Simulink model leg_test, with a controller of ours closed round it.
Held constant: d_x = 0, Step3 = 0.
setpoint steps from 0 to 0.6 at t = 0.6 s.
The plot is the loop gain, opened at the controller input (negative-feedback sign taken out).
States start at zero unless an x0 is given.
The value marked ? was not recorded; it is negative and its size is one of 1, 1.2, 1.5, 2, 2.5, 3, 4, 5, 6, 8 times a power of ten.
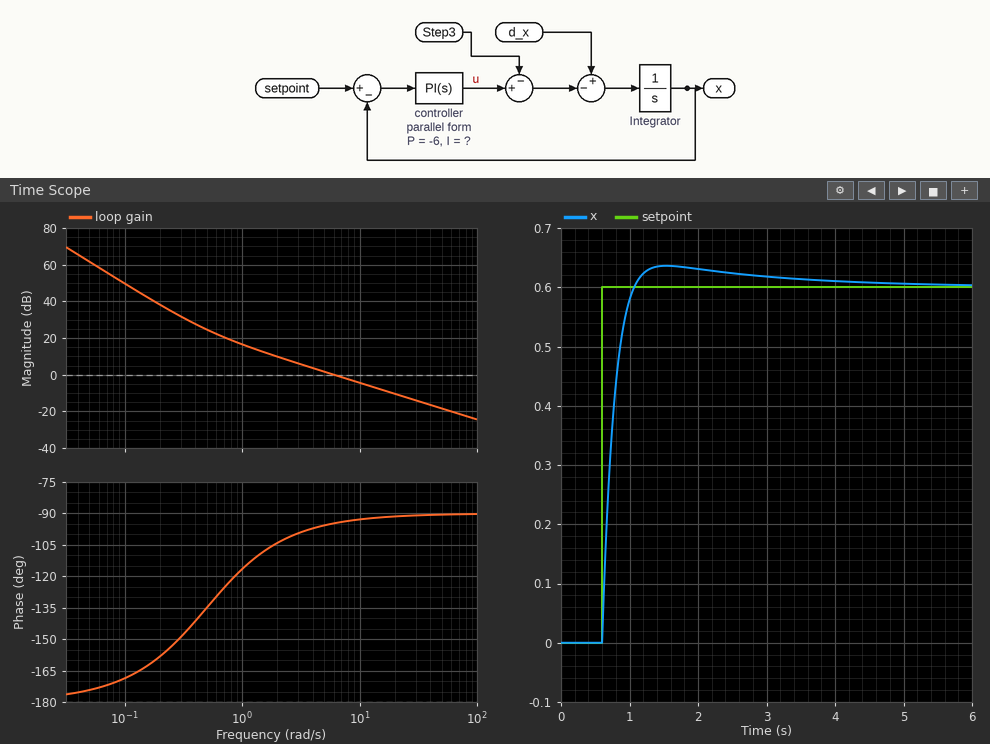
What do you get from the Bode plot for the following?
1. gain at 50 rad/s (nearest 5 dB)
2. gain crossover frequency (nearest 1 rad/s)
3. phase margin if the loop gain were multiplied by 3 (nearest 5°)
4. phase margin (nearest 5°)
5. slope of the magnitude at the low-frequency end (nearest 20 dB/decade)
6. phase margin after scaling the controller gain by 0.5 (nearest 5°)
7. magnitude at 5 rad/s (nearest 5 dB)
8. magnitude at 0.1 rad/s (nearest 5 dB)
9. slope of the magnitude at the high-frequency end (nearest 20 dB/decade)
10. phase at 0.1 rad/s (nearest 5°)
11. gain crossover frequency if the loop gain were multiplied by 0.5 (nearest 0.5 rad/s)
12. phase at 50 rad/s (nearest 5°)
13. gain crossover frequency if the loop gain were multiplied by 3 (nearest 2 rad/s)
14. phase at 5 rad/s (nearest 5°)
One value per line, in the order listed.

-20 dB
6 rad/s
90°
85°
-40 dB/decade
80°
0 dB
50 dB
-20 dB/decade
-170°
3.0 rad/s
-90°
18 rad/s
-95°
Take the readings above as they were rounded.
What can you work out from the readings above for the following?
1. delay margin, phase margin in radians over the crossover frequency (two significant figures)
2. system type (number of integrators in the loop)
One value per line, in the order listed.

0.25 s
2
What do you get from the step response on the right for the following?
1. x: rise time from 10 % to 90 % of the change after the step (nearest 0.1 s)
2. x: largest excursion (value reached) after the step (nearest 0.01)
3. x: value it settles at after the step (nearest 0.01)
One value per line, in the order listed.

0.3 s
0.64
0.60
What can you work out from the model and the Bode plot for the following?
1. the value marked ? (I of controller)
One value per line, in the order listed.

-3
